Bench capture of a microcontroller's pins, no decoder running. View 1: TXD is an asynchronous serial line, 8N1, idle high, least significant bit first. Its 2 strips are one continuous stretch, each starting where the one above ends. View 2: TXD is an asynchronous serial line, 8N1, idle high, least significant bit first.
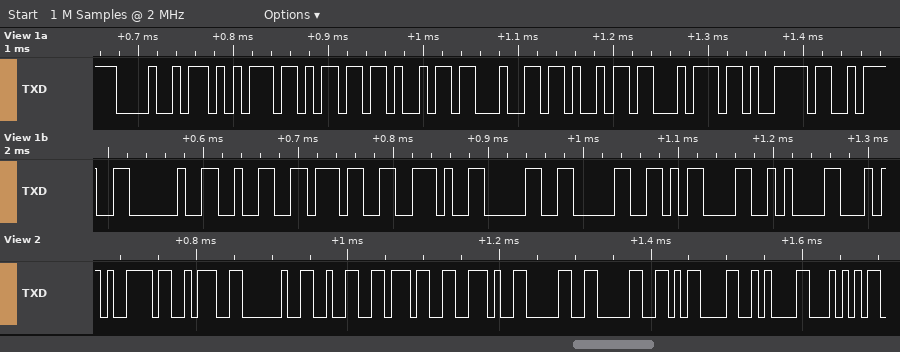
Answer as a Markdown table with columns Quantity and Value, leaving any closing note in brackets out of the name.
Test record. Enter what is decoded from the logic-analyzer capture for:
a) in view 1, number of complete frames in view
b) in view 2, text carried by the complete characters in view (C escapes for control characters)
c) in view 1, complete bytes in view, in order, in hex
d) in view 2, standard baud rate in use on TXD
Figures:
| Quantity | Value |
|---|---|
| in view 1, number of complete frames in view | 17 |
| in view 2, text carried by the complete characters in view | "y: 27.00\r\nT" |
| in view 1, complete bytes in view, in order, in hex | 48 75 6D 69 64 69 74 79 3A 20 32 37 2E 30 30 0D 0A |
| in view 2, standard baud rate in use on TXD | 115200 baud |
